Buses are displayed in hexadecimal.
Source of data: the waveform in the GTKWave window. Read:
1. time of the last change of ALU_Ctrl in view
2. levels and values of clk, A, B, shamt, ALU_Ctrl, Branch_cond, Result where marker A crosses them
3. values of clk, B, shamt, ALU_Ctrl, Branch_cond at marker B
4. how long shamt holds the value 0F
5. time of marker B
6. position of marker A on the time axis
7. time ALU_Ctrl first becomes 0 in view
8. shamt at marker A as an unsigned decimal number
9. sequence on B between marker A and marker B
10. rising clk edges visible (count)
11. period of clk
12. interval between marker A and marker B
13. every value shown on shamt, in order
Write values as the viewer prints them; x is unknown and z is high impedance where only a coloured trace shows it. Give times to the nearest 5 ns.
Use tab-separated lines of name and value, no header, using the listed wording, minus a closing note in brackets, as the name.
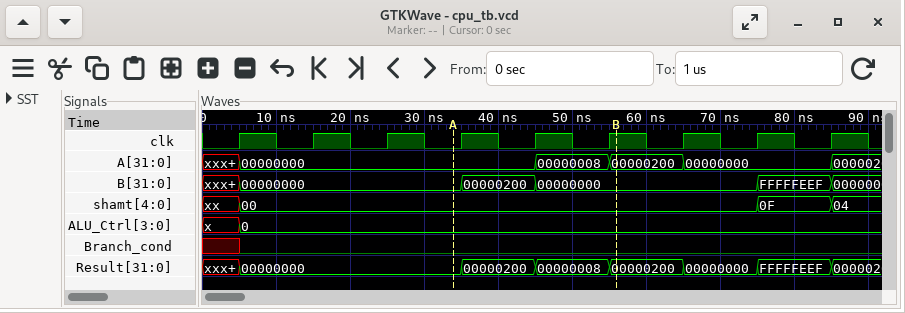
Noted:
time of the last change of ALU_Ctrl in view	5 ns
levels and values of clk, A, B, shamt, ALU_Ctrl, Branch_cond, Result where marker A crosses them	clk=0, A=00000000, B=00000000, shamt=00, ALU_Ctrl=0, Branch_cond=0, Result=00000000
values of clk, B, shamt, ALU_Ctrl, Branch_cond at marker B	clk=1, B=00000000, shamt=00, ALU_Ctrl=0, Branch_cond=0
how long shamt holds the value 0F	10 ns
time of marker B	55 ns
position of marker A on the time axis	35 ns
time ALU_Ctrl first becomes 0 in view	5 ns
shamt at marker A as an unsigned decimal number	0
sequence on B between marker A and marker B	00000000, 00000200, 00000000
rising clk edges visible	9
period of clk	10 ns
interval between marker A and marker B	20 ns
every value shown on shamt, in order	xx, 00, 0F, 04
